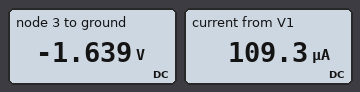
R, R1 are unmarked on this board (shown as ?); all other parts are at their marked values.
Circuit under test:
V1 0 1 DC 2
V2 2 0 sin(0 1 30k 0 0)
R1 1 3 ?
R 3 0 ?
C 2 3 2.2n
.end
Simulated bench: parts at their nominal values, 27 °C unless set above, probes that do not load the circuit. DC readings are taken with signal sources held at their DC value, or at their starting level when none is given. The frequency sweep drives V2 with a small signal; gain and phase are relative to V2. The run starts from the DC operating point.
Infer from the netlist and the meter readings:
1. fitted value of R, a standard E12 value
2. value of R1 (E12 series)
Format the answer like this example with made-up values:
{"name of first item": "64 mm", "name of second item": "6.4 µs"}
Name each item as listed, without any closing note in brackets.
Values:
{"fitted value of R, a standard E12 value": "15 kΩ", "value of R1": "3.3 kΩ"}
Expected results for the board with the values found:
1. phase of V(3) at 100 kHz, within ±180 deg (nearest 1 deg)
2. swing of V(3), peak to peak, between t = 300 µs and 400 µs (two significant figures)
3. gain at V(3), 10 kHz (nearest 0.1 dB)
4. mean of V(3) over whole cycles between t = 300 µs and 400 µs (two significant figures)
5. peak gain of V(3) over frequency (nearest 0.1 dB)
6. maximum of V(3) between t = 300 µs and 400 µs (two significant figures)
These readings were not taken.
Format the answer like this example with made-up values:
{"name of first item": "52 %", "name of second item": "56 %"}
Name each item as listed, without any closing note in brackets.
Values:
{"phase of V(3) at 100 kHz, within ±180 deg": "15 deg", "swing of V(3), peak to peak, between t = 300 µs and 400 µs": "1.5 V", "gain at V(3), 10 kHz": "-9.1 dB", "mean of V(3) over whole cycles between t = 300 µs and 400 µs": "-1.6 V", "peak gain of V(3) over frequency": "0 dB", "maximum of V(3) between t = 300 µs and 400 µs": "-890 mV"}
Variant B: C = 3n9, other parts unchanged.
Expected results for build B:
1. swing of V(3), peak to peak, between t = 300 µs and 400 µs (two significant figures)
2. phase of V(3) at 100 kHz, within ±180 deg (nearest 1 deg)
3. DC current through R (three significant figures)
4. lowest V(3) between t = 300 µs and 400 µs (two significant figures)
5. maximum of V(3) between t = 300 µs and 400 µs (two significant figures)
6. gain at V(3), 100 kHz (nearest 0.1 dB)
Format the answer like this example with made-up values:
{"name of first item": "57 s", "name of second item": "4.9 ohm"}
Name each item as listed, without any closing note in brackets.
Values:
{"swing of V(3), peak to peak, between t = 300 µs and 400 µs": "1.8 V", "phase of V(3) at 100 kHz, within ±180 deg": "9 deg", "DC current through R": "109 µA", "lowest V(3) between t = 300 µs and 400 µs": "-2.5 V", "maximum of V(3) between t = 300 µs and 400 µs": "-750 mV", "gain at V(3), 100 kHz": "-0.1 dB"}
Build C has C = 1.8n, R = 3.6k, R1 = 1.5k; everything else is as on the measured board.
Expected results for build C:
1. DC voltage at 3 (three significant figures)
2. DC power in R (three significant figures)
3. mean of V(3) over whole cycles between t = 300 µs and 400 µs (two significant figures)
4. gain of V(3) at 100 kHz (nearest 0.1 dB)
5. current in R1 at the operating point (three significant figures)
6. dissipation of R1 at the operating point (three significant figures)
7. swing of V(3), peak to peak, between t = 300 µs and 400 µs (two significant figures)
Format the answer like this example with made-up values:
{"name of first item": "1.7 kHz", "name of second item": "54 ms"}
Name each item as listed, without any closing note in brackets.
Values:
{"DC voltage at 3": "-1.41 V", "DC power in R": "554 µW", "mean of V(3) over whole cycles between t = 300 µs and 400 µs": "-1.4 V", "gain of V(3) at 100 kHz": "-2.3 dB", "current in R1 at the operating point": "392 µA", "dissipation of R1 at the operating point": "231 µW", "swing of V(3), peak to peak, between t = 300 µs and 400 µs": "680 mV"}
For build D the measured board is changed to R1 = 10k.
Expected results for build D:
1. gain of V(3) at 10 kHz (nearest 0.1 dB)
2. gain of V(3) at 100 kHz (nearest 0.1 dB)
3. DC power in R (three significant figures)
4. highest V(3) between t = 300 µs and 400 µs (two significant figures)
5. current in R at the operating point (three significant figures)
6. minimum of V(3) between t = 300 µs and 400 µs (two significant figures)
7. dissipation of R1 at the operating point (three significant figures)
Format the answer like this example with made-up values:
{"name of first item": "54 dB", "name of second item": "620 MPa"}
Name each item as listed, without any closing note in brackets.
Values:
{"gain of V(3) at 10 kHz": "-3.9 dB", "gain of V(3) at 100 kHz": "-0.1 dB", "DC power in R": "96.0 µW", "highest V(3) between t = 300 µs and 400 µs": "-270 mV", "current in R at the operating point": "80.0 µA", "minimum of V(3) between t = 300 µs and 400 µs": "-2.1 V", "dissipation of R1 at the operating point": "64.0 µW"}
